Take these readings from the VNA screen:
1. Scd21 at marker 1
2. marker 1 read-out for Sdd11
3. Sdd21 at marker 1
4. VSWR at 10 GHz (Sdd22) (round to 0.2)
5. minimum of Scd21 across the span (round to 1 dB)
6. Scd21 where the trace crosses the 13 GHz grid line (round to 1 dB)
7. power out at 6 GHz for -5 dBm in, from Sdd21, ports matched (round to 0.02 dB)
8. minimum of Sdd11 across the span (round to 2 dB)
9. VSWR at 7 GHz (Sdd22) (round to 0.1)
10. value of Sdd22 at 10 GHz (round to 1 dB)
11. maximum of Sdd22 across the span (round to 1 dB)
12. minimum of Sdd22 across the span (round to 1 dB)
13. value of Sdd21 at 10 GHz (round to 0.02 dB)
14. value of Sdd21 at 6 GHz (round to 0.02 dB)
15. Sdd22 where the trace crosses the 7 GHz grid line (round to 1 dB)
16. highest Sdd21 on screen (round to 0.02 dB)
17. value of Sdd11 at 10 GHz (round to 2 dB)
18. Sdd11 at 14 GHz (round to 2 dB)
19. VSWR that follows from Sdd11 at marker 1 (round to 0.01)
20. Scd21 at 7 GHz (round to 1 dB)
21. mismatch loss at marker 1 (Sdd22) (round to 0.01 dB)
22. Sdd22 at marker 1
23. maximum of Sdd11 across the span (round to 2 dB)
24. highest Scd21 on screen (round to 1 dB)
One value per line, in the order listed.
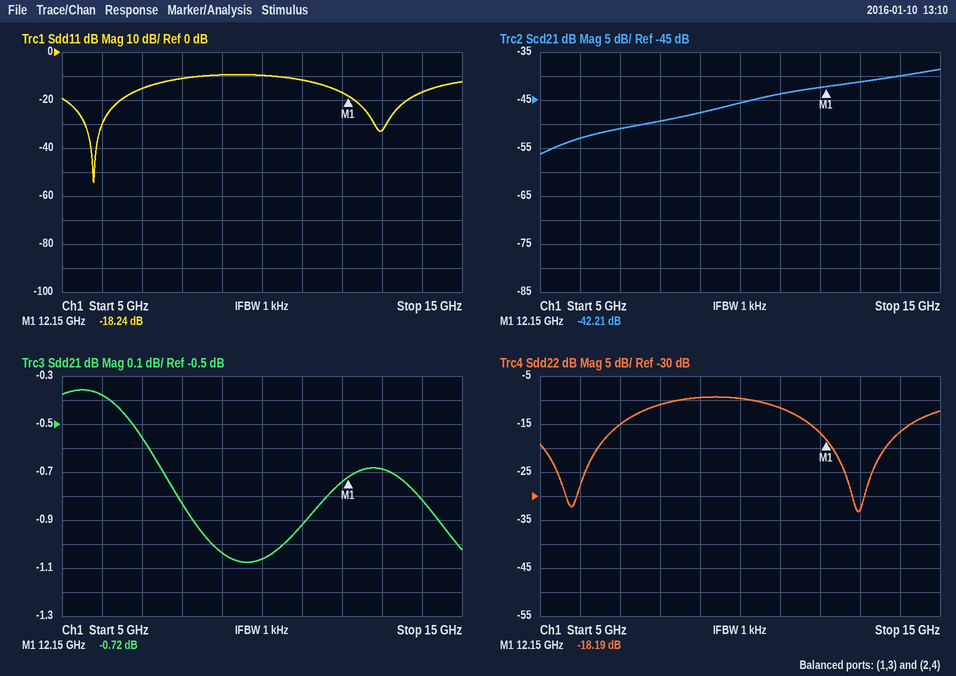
-42.21 dB
-18.24 dB
-0.72 dB
2.0
-56 dB
-41 dB
-5.38 dBm
-54 dB
1.4
-10 dB
-9 dB
-33 dB
-1.06 dB
-0.38 dB
-15 dB
-0.36 dB
-10 dB
-16 dB
1.28
-51 dB
0.07 dB
-18.19 dB
-10 dB
-39 dB
